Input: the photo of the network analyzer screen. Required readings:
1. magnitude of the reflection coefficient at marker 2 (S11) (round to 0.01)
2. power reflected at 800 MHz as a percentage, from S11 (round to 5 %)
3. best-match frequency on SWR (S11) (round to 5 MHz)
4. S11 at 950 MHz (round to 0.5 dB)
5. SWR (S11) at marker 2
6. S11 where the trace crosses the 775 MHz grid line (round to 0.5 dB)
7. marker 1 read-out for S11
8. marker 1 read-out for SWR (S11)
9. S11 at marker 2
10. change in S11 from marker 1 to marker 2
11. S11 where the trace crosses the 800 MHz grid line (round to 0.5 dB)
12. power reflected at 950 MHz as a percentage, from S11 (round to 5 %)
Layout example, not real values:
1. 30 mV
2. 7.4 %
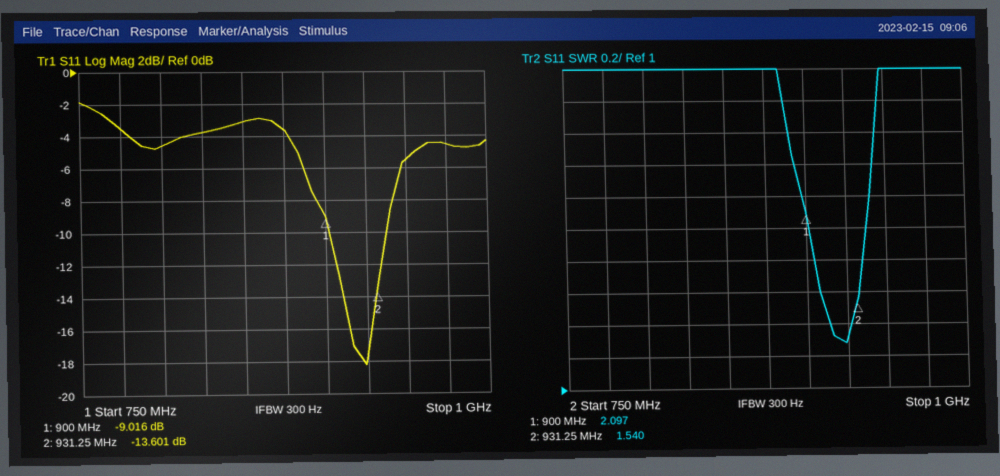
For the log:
1. 0.21
2. 35 %
3. 925 MHz
4. -5.5 dB
5. 1.540
6. -3.5 dB
7. -9.016 dB
8. 2.097
9. -13.601 dB
10. -4.585 dB
11. -4.5 dB
12. 30 %
